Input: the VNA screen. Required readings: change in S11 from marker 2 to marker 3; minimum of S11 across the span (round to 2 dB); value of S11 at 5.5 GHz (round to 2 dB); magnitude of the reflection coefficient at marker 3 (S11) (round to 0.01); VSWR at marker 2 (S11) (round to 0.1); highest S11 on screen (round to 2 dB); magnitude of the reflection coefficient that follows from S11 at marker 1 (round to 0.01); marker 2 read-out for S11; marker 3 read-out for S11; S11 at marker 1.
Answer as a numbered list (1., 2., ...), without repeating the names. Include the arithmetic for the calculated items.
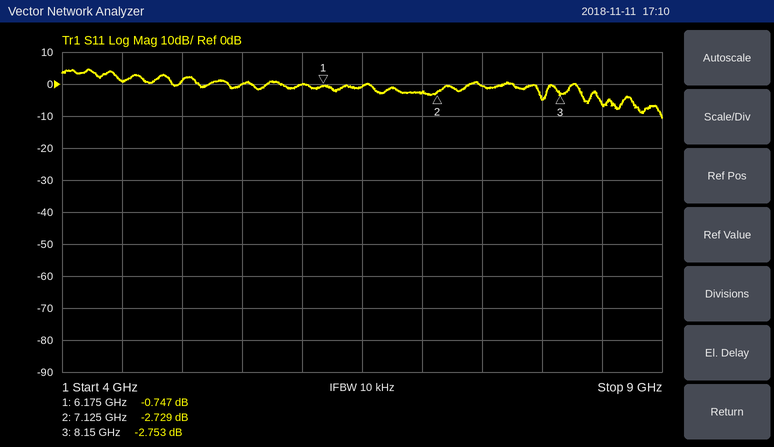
1. -2.753 − (-2.729) = -0.024 dB
2. -10 dB
3. 0 dB
4. 10^(-2.753/20) ≈ 0.73
5. (1 + 0.7304)/(1 − 0.7304) ≈ 6.4
6. 4 dB
7. 10^(-0.747/20) ≈ 0.92
8. -2.729 dB
9. -2.753 dB
10. -0.747 dB
